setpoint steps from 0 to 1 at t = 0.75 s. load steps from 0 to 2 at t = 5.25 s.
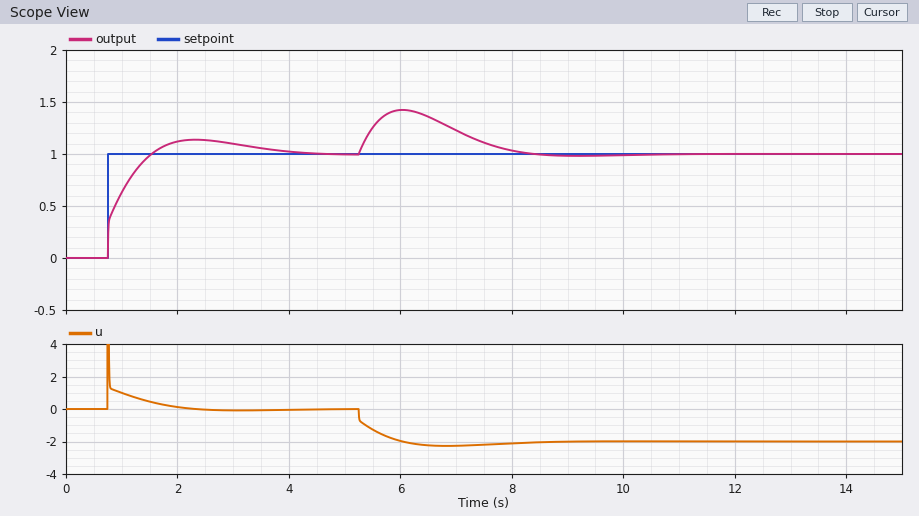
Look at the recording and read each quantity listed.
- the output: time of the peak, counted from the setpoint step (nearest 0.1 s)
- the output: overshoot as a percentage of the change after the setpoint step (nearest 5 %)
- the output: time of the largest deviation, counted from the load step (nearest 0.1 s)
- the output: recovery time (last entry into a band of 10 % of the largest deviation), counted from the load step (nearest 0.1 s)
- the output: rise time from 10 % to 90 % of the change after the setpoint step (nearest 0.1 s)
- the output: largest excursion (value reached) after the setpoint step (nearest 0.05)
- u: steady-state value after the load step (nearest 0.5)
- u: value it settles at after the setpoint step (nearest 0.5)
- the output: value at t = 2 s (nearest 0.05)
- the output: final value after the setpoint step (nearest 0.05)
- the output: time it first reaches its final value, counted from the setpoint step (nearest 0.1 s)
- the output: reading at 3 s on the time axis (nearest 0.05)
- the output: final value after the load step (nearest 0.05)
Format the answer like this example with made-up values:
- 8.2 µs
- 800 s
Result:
- 1.6 s
- 15 %
- 0.8 s
- 2.7 s
- 0.6 s
- 1.15
- -2.0
- 0.0
- 1.10
- 1.00
- 0.8 s
- 1.10
- 1.00
